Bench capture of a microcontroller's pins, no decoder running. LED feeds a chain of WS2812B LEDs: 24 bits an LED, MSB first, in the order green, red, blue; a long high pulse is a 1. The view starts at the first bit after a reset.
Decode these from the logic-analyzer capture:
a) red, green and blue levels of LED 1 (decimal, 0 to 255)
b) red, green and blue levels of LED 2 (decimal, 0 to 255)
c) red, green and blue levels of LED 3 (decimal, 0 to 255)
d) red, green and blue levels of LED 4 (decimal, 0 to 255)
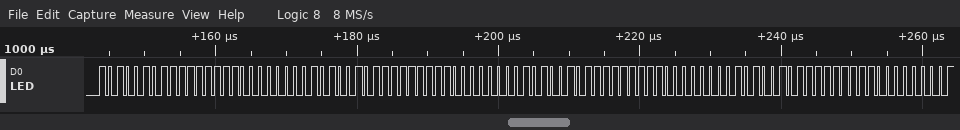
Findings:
255, 165, 0
255, 165, 0
255, 165, 0
255, 165, 0
